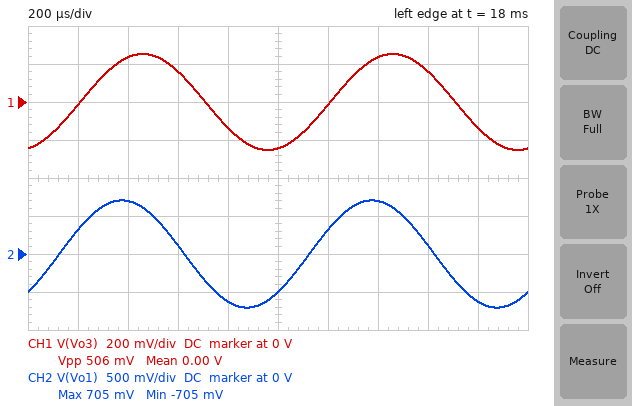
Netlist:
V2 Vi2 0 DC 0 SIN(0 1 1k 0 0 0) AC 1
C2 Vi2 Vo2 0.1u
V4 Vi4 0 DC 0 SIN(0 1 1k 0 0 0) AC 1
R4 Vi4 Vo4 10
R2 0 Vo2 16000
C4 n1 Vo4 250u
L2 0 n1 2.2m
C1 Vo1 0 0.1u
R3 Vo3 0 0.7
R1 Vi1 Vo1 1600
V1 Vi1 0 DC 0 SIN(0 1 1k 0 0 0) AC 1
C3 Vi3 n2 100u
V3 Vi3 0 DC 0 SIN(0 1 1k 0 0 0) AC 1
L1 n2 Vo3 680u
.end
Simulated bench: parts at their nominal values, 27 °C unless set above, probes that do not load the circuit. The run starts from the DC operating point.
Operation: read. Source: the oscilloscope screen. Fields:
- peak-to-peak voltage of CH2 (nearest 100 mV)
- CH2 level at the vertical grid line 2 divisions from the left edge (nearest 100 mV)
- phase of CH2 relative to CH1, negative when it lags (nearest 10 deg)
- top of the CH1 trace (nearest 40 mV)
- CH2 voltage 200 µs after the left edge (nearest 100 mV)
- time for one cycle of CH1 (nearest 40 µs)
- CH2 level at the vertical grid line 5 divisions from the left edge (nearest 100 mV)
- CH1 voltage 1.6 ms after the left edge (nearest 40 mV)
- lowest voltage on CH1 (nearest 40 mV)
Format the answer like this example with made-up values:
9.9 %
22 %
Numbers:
1.4 V
700 mV
30 deg
240 mV
300 mV
1.00 ms
-500 mV
160 mV
-240 mV
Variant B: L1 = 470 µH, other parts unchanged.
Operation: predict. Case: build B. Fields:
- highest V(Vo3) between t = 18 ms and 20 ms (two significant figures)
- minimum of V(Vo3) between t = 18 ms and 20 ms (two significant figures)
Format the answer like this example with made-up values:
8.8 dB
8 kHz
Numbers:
460 mV
-460 mV
